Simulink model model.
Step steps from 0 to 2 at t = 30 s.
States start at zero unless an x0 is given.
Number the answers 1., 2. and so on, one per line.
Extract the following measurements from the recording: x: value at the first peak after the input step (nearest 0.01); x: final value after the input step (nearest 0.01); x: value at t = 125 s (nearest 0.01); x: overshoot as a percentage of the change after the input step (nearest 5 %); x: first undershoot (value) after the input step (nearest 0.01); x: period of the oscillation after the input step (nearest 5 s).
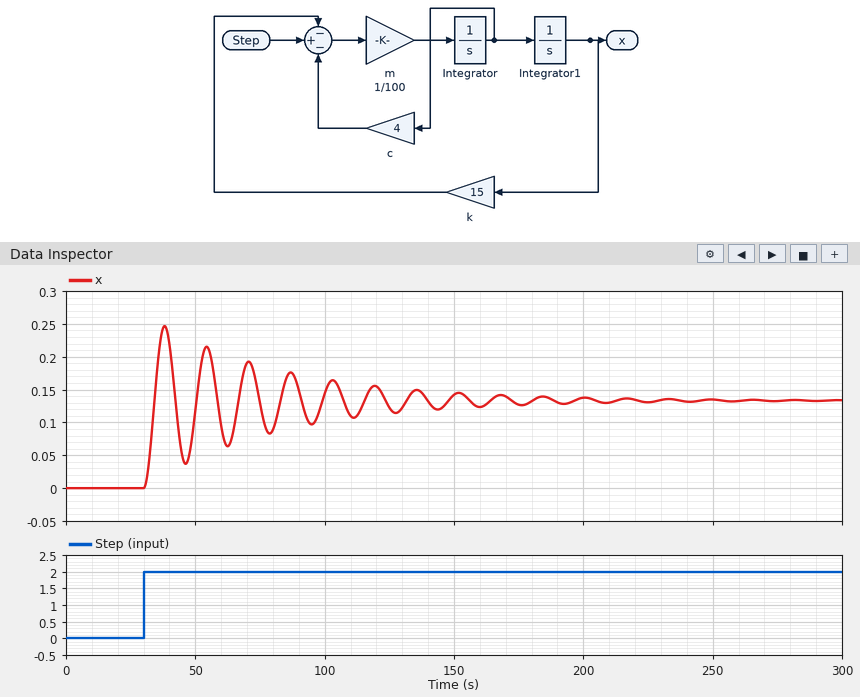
1. 0.25
2. 0.13
3. 0.12
4. 85 %
5. 0.04
6. 15 s
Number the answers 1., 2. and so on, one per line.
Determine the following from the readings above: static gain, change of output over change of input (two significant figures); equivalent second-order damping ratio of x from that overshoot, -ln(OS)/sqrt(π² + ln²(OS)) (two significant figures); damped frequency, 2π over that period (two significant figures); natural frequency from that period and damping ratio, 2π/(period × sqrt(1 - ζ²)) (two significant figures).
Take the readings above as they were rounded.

1. 0.065
2. 0.052
3. 0.42 rad/s
4. 0.42 rad/s
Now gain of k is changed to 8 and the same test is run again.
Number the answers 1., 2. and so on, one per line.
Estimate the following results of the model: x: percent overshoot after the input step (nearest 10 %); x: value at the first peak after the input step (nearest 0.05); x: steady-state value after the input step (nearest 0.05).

1. 80 %
2. 0.45
3. 0.25
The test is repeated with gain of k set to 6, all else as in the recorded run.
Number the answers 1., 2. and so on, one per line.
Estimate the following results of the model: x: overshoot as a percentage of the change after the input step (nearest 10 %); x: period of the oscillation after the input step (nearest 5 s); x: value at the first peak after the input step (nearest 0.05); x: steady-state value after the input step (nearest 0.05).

1. 80 %
2. 25 s
3. 0.60
4. 0.35
